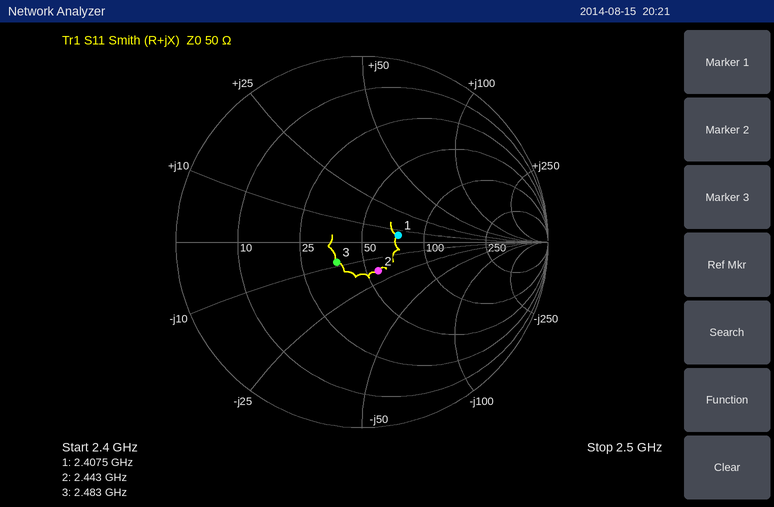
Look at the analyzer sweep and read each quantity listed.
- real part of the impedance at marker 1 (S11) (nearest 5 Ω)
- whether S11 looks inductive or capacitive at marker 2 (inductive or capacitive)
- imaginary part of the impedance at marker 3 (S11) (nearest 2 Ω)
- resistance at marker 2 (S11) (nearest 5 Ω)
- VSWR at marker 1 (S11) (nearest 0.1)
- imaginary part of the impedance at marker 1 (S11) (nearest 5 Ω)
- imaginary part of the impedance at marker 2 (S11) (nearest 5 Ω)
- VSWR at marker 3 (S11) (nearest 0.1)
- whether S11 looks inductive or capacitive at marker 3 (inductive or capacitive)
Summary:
75 Ω
capacitive
-8 Ω
55 Ω
1.5
+5 Ω
-20 Ω
1.4
capacitive
